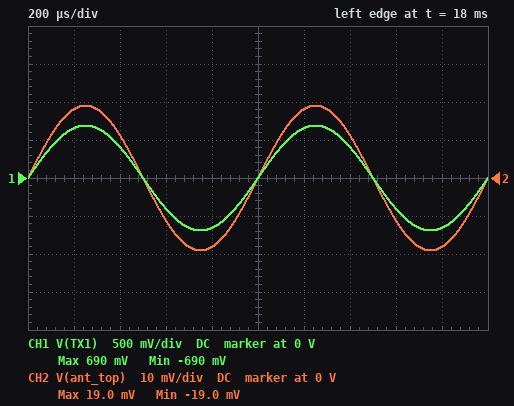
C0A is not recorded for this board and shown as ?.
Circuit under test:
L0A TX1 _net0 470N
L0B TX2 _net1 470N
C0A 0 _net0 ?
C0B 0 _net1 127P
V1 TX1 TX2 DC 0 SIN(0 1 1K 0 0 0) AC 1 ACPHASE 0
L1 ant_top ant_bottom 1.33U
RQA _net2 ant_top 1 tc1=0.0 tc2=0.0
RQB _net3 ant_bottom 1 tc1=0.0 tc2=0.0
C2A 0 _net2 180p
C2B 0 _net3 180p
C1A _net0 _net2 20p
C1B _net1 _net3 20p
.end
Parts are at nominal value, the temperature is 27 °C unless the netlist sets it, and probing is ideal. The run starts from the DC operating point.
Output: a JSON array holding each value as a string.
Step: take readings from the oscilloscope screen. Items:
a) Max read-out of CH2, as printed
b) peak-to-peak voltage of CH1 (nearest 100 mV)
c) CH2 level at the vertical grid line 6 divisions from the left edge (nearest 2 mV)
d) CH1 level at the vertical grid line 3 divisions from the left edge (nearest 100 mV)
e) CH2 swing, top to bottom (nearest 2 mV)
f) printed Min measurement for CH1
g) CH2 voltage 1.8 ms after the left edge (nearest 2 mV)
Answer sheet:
["19.0 mV", "1.4 V", "18 mV", "-400 mV", "38 mV", "-690 mV", "-18 mV"]
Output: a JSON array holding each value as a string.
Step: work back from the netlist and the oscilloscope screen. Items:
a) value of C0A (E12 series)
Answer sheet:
["47 pF"]
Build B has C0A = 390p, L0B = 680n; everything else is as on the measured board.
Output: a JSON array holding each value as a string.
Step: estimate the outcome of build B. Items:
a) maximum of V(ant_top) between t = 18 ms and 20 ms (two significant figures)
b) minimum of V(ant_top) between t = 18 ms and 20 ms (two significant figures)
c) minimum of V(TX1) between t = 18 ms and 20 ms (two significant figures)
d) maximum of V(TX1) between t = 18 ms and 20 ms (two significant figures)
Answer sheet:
["24 mV", "-24 mV", "-260 mV", "260 mV"]
